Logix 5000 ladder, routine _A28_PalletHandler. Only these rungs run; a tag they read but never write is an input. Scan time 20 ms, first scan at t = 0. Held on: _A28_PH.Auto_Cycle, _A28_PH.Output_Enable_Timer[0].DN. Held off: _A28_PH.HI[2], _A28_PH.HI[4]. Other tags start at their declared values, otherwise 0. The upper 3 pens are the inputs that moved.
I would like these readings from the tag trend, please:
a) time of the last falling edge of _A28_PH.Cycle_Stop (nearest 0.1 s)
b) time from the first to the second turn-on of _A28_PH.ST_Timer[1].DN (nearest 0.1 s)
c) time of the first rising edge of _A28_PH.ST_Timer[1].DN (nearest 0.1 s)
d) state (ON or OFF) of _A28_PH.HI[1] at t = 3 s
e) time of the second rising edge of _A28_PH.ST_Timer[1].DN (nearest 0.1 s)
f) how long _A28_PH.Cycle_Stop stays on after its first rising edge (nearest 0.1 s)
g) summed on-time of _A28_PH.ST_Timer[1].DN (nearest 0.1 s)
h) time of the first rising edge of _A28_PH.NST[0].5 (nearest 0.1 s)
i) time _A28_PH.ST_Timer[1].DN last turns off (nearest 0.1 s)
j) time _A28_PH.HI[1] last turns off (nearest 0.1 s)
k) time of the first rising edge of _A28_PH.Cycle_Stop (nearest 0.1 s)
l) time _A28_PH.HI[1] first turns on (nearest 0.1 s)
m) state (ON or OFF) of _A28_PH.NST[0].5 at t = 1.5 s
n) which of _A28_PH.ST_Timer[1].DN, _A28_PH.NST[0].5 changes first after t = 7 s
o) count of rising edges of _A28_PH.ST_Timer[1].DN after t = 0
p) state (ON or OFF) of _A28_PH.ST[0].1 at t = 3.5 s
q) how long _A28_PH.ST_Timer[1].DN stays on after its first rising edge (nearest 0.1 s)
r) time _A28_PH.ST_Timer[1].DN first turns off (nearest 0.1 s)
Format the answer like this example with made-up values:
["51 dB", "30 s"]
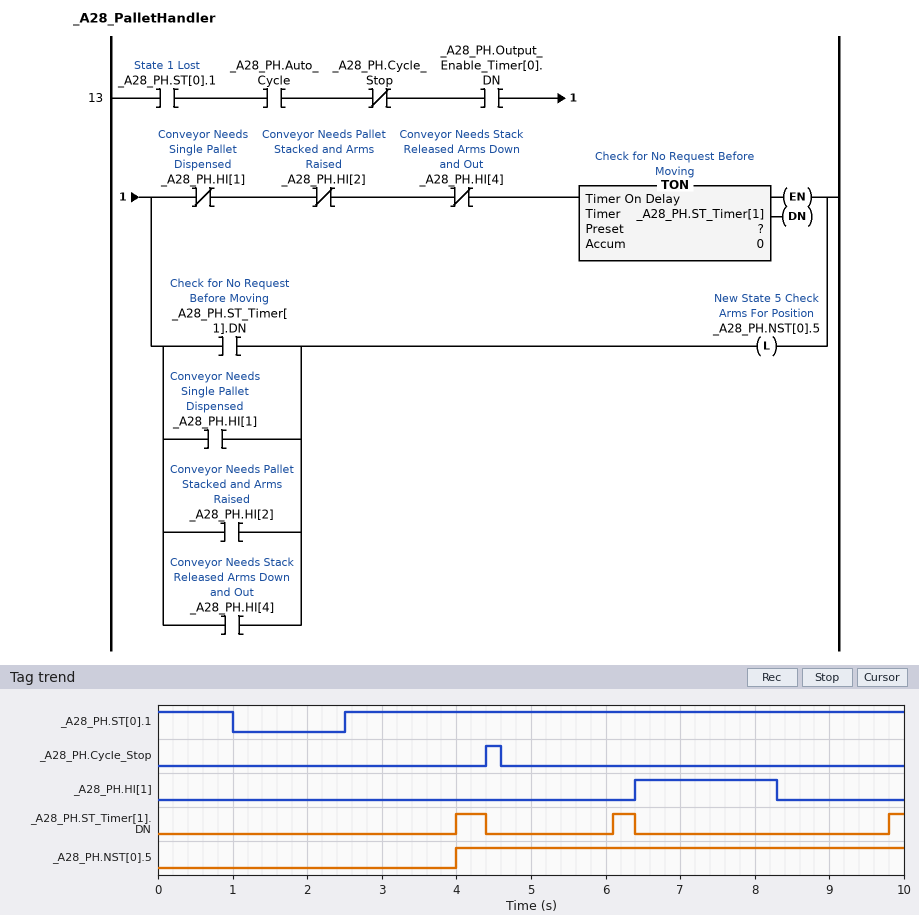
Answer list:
["4.6 s", "2.1 s", "4.0 s", "OFF", "6.1 s", "0.2 s", "0.9 s", "4.0 s", "6.4 s", "8.3 s", "4.4 s", "6.4 s", "OFF", "_A28_PH.ST_Timer[1].DN", "3", "ON", "0.4 s", "4.4 s"]
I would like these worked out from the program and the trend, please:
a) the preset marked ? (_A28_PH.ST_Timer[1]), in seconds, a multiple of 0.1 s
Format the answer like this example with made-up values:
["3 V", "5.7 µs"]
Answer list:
["1.5 s"]
